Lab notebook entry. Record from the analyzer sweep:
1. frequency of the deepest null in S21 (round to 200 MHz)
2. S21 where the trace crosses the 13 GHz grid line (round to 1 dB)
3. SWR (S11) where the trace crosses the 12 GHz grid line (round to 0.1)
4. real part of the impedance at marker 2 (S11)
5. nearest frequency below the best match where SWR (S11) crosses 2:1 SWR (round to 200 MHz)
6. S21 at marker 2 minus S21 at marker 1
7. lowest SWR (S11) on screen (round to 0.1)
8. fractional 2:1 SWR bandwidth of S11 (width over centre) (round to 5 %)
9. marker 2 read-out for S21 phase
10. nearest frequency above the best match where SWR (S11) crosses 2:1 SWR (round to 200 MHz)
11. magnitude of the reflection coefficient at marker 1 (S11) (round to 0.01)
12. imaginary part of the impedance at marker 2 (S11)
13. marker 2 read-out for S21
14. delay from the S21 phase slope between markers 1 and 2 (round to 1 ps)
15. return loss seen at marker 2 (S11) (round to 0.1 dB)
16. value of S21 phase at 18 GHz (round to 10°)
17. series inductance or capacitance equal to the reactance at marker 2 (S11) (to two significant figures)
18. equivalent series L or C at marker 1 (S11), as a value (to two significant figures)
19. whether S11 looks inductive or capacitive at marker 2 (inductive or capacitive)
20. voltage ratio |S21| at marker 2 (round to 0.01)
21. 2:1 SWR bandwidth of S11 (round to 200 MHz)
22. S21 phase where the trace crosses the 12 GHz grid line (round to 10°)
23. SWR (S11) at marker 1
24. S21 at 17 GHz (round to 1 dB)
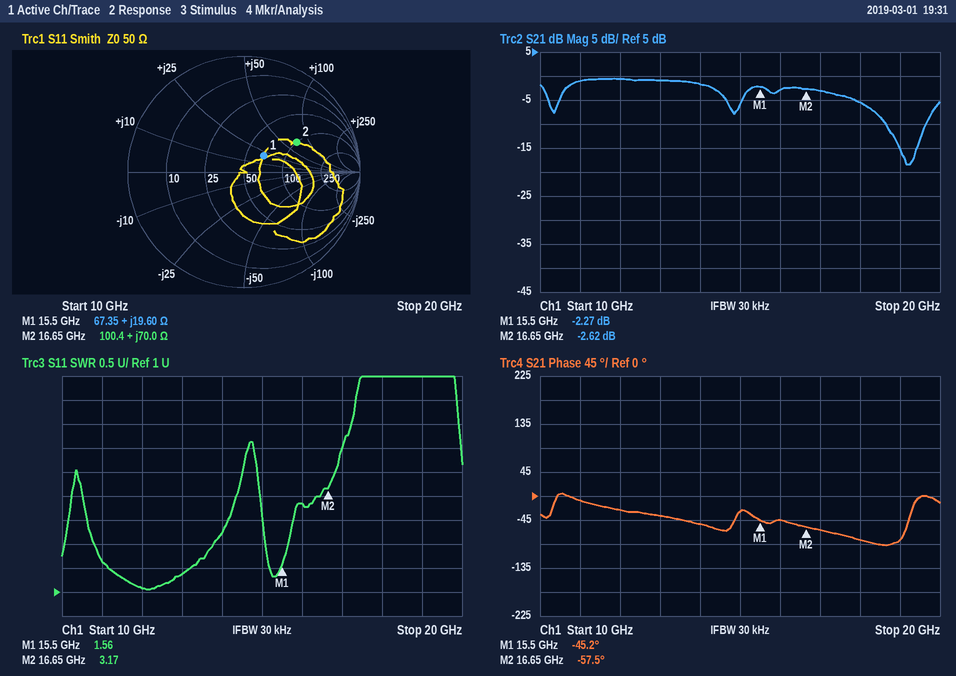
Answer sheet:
19.2 GHz
-1 dB
1.1
100.4 Ω
10.8 GHz
-0.35 dB
1.1
25 %
-57.5°
13.8 GHz
0.22
+70.0 Ω
-2.62 dB
30 ps
5.7 dB
-80°
670 pH
200 pH
inductive
0.74
3.0 GHz
-30°
1.56
-3 dB
